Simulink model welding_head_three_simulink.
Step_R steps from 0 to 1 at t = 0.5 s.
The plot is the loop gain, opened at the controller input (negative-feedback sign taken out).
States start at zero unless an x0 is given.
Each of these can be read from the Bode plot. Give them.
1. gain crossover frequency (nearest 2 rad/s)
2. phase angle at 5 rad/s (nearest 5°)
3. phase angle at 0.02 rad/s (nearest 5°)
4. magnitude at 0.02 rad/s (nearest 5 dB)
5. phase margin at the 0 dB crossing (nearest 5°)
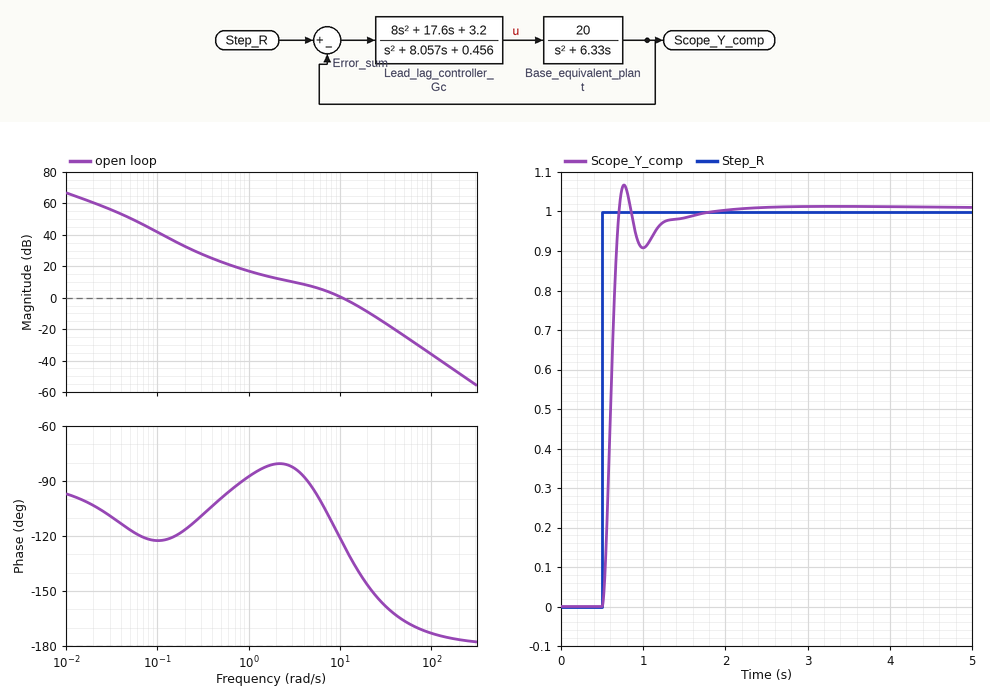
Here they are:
10 rad/s
-95°
-105°
60 dB
55°
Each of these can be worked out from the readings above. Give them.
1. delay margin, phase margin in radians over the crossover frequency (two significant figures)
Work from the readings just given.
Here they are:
0.096 s
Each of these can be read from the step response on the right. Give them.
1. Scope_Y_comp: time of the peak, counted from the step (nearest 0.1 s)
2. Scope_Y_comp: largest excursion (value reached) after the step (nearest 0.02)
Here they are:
0.3 s
1.06
